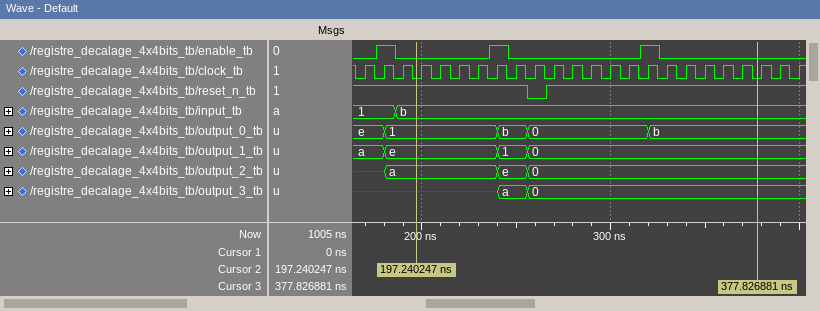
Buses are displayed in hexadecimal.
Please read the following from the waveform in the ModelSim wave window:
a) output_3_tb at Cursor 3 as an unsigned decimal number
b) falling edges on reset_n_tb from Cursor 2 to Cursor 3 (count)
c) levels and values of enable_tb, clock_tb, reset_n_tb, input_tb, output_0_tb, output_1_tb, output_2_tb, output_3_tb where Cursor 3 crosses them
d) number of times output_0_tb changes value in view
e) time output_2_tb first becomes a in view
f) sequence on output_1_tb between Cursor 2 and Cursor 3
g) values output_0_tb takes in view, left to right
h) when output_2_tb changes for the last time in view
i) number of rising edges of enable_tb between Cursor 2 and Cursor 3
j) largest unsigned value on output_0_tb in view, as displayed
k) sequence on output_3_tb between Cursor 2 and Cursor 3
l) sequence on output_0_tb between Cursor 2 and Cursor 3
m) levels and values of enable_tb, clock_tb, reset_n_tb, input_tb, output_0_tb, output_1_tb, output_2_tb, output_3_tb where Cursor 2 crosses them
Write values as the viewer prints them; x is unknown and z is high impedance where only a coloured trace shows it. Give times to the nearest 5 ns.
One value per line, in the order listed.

0
1
enable_tb=0, clock_tb=0, reset_n_tb=1, input_tb=b, output_0_tb=b, output_1_tb=0, output_2_tb=0, output_3_tb=0
4
180 ns
e, 1, 0
e, 1, b, 0, b
255 ns
2
e
x, a, 0
1, b, 0, b
enable_tb=0, clock_tb=0, reset_n_tb=1, input_tb=b, output_0_tb=1, output_1_tb=e, output_2_tb=a, output_3_tb=x
